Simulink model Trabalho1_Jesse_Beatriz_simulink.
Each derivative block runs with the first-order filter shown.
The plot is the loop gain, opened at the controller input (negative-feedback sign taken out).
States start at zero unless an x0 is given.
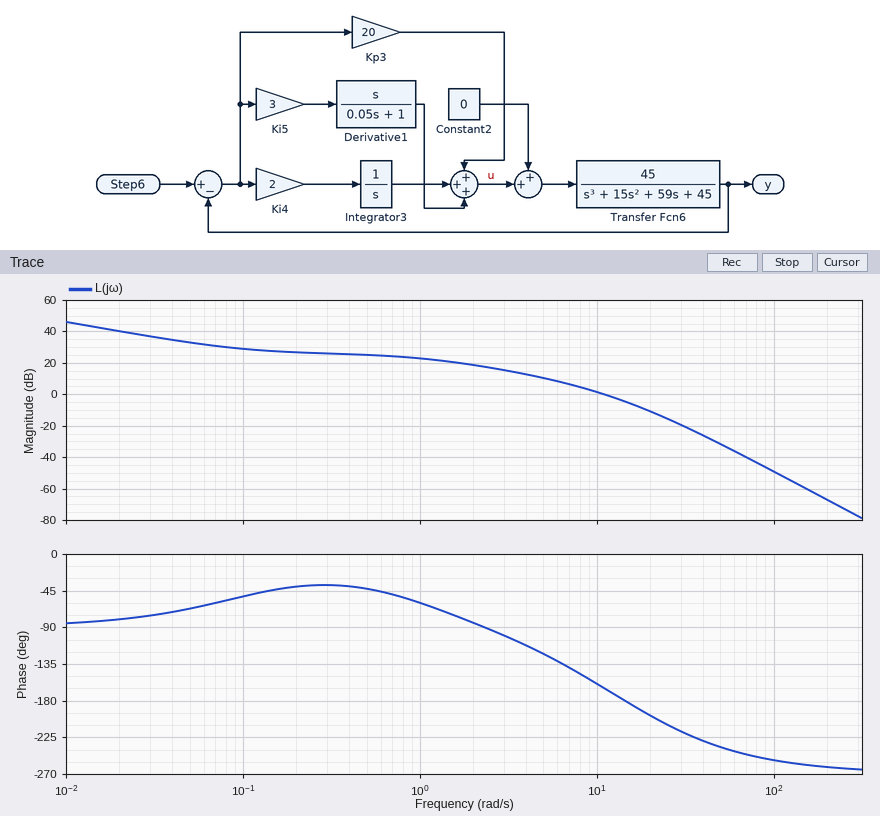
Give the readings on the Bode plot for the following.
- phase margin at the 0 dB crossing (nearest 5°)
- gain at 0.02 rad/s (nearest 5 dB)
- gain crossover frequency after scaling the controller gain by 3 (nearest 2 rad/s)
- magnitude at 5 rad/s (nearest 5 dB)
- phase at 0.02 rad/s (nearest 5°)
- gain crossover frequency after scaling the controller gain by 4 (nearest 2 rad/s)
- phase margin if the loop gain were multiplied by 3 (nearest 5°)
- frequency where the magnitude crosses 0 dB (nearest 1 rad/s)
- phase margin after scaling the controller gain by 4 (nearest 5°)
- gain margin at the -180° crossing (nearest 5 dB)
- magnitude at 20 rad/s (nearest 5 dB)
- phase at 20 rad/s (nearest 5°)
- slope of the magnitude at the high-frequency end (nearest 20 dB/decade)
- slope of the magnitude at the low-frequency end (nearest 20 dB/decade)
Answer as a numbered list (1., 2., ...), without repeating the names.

1. 15°
2. 40 dB
3. 18 rad/s
4. 10 dB
5. -80°
6. 22 rad/s
7. -15°
8. 11 rad/s
9. -20°
10. 5 dB
11. -10 dB
12. -200°
13. -60 dB/decade
14. -20 dB/decade
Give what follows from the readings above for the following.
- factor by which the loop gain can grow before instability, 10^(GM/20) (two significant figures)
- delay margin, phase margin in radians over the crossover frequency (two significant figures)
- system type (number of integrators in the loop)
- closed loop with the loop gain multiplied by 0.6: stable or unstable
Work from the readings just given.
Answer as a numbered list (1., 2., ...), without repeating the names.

1. 1.8
2. 0.024 s
3. 1
4. stable
